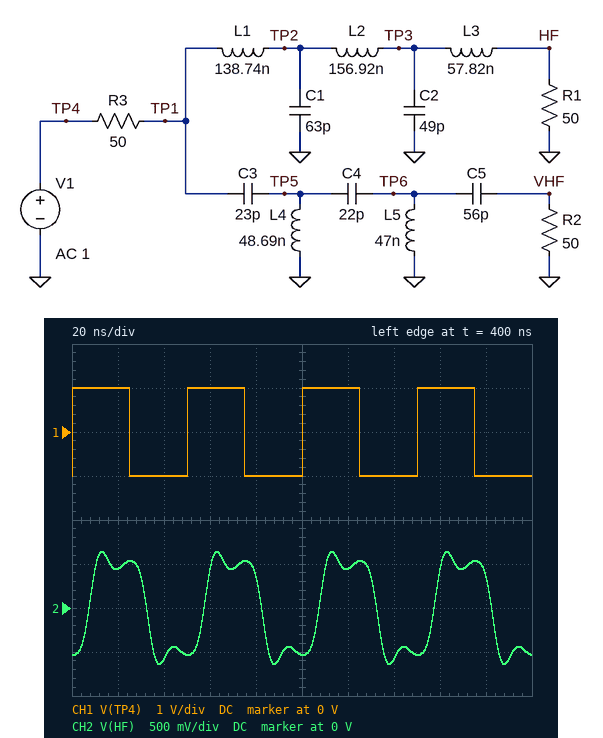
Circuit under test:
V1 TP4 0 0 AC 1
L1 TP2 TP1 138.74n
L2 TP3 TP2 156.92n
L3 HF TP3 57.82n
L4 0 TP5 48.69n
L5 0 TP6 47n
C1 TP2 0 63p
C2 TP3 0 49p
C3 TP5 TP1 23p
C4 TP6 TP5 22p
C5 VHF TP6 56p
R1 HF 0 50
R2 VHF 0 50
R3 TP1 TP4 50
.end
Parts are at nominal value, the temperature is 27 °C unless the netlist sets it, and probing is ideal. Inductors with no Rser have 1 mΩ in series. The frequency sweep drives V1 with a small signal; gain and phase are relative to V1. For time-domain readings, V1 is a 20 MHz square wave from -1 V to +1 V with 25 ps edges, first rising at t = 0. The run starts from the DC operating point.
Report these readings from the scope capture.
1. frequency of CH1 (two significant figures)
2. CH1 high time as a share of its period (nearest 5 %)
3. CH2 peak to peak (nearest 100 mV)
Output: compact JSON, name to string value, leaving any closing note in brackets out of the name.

{"frequency of CH1": "20 MHz", "CH1 high time as a share of its period": "50 %", "CH2 peak to peak": "1.3 V"}
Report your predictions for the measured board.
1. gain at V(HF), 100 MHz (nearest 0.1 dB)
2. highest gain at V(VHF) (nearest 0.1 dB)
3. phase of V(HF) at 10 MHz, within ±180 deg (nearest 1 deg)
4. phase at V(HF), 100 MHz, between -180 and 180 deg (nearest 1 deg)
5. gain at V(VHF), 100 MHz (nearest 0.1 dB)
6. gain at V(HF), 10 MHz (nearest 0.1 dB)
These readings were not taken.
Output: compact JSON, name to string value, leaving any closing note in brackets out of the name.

{"gain at V(HF), 100 MHz": "-16.4 dB", "highest gain at V(VHF)": "-6.0 dB", "phase of V(HF) at 10 MHz, within ±180 deg": "-25 deg", "phase at V(HF), 100 MHz, between -180 and 180 deg": "44 deg", "gain at V(VHF), 100 MHz": "-6.8 dB", "gain at V(HF), 10 MHz": "-6.0 dB"}
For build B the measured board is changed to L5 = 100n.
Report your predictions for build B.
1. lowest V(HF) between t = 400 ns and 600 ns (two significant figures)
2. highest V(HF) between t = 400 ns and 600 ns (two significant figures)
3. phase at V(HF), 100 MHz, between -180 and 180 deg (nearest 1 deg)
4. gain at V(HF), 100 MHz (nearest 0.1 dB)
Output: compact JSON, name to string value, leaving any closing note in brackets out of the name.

{"lowest V(HF) between t = 400 ns and 600 ns": "-660 mV", "highest V(HF) between t = 400 ns and 600 ns": "660 mV", "phase at V(HF), 100 MHz, between -180 and 180 deg": "25 deg", "gain at V(HF), 100 MHz": "-13.4 dB"}
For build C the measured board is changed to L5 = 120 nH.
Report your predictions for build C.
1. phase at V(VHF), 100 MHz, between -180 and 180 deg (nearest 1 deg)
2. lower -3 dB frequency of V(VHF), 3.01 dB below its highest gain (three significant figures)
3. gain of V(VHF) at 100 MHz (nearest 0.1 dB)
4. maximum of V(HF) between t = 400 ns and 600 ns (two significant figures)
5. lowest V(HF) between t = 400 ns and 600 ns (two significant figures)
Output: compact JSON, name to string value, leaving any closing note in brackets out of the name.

{"phase at V(VHF), 100 MHz, between -180 and 180 deg": "-144 deg", "lower -3 dB frequency of V(VHF), 3.01 dB below its highest gain": "94.2 MHz", "gain of V(VHF) at 100 MHz": "-7.4 dB", "maximum of V(HF) between t = 400 ns and 600 ns": "660 mV", "lowest V(HF) between t = 400 ns and 600 ns": "-660 mV"}
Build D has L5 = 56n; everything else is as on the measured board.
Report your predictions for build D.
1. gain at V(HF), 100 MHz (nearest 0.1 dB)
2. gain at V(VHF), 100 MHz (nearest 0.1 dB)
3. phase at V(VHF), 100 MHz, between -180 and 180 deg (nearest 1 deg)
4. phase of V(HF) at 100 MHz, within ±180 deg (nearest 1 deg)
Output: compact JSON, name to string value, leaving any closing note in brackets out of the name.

{"gain at V(HF), 100 MHz": "-15.1 dB", "gain at V(VHF), 100 MHz": "-6.7 dB", "phase at V(VHF), 100 MHz, between -180 and 180 deg": "-121 deg", "phase of V(HF) at 100 MHz, within ±180 deg": "39 deg"}
